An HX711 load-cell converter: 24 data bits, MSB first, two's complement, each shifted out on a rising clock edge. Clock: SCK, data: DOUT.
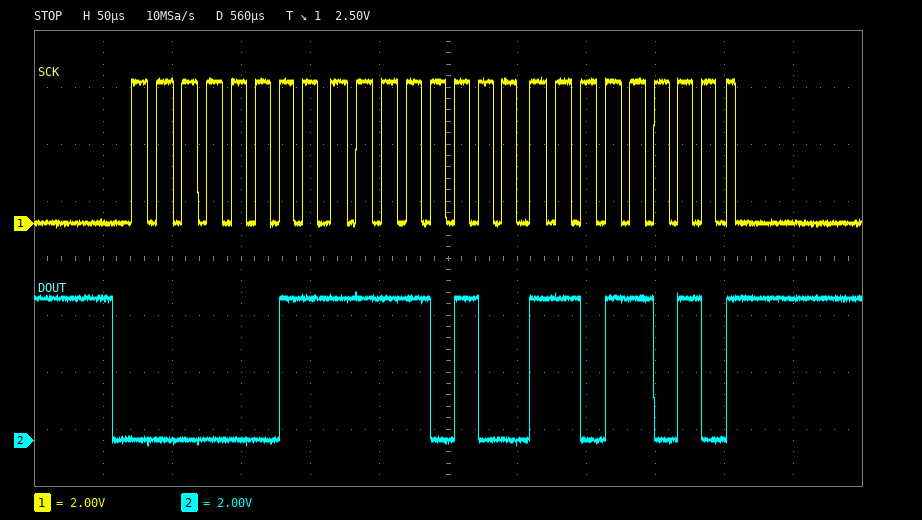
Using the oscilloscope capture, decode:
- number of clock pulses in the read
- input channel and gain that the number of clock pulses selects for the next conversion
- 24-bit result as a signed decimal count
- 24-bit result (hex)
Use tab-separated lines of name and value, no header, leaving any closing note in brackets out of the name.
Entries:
number of clock pulses in the read	25
input channel and gain that the number of clock pulses selects for the next conversion	channel A, gain 128
24-bit result as a signed decimal count	259290
24-bit result	0x03F4DA
